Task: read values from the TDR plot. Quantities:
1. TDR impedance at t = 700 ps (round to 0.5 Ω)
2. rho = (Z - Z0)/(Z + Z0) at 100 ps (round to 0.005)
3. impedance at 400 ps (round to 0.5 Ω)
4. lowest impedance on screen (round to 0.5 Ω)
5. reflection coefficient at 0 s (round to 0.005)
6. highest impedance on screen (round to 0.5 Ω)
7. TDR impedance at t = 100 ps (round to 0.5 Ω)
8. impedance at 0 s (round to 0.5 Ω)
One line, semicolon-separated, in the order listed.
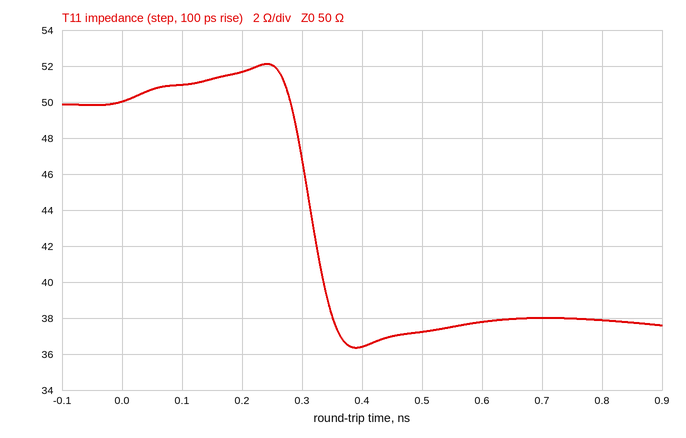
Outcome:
38.0 Ω; +0.010; 36.5 Ω; 36.5 Ω; 0.000; 52.0 Ω; 51.0 Ω; 50.0 Ω
